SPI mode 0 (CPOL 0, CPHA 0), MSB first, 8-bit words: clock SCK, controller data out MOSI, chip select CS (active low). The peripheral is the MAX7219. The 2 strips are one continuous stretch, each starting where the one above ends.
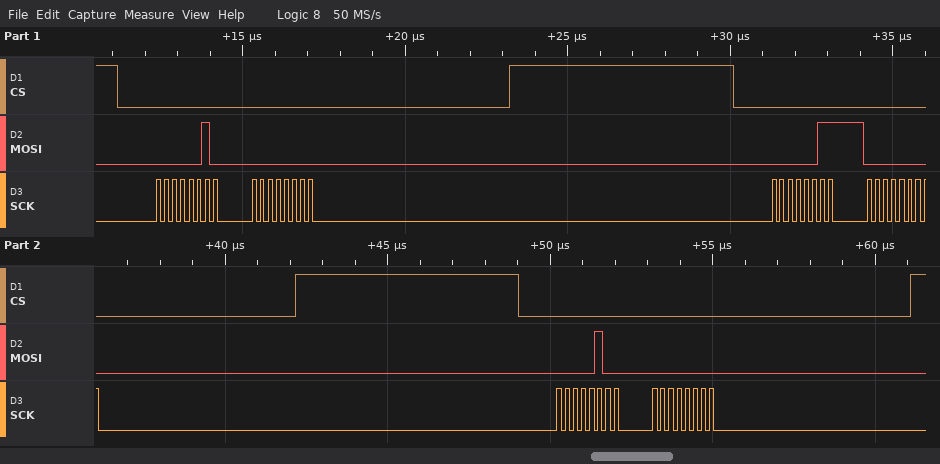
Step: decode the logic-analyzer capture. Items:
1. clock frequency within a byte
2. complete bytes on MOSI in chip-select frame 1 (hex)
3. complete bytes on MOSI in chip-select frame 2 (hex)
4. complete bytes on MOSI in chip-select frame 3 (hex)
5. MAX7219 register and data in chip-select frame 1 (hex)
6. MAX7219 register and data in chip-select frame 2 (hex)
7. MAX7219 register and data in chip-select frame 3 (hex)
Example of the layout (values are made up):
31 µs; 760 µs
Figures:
4 MHz; 02 00; 03 00; 04 00; register 0x2, data 0x00; register 0x3, data 0x00; register 0x4, data 0x00
